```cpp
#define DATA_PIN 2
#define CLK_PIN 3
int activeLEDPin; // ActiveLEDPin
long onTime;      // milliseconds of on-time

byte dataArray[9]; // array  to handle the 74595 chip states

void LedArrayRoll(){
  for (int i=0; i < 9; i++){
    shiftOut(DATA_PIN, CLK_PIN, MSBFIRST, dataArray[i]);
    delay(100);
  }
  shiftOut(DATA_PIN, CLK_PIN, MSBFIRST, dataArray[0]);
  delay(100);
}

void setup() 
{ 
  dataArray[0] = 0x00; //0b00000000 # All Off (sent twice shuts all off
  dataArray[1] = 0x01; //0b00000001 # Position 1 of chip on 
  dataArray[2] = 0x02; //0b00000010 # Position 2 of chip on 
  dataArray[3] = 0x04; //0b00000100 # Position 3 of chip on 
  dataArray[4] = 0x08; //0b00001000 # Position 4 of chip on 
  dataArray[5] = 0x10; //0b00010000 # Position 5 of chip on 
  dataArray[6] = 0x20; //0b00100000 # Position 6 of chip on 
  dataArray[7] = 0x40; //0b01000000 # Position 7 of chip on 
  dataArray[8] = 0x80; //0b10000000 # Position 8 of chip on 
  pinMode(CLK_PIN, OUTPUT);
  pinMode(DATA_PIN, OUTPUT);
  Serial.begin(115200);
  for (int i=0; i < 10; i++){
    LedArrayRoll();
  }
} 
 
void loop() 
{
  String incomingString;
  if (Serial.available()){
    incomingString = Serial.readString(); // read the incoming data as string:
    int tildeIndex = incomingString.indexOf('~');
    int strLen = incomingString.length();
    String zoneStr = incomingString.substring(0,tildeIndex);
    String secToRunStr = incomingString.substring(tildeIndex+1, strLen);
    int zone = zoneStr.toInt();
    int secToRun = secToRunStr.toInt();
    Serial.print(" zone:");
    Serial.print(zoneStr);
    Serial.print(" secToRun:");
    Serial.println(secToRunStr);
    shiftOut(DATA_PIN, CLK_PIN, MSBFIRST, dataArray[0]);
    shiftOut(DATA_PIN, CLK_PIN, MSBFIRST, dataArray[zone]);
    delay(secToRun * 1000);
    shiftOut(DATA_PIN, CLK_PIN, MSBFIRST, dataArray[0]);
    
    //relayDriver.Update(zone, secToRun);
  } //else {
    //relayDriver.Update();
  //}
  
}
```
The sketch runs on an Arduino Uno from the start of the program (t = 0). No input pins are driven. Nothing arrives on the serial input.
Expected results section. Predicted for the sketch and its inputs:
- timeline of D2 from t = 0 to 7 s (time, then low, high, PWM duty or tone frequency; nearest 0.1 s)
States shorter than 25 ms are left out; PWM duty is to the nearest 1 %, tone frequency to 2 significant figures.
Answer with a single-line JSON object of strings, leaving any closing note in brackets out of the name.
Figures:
{"timeline of D2 from t = 0 to 7 s": "0 s low; 0.1 s high; 0.2 s low; 1.1 s high; 1.2 s low; 2.1 s high; 2.2 s low; 3.1 s high; 3.2 s low; 4.1 s high; 4.2 s low; 5.1 s high; 5.2 s low; 6.1 s high; 6.2 s low"}
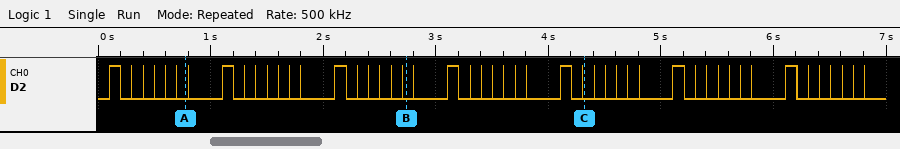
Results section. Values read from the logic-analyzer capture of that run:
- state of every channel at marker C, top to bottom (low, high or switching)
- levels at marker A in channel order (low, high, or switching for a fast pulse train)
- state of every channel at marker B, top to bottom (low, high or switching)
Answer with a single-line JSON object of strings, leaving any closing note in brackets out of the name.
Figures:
{"state of every channel at marker C, top to bottom": "D2 low", "levels at marker A in channel order": "D2 low", "state of every channel at marker B, top to bottom": "D2 low"}
